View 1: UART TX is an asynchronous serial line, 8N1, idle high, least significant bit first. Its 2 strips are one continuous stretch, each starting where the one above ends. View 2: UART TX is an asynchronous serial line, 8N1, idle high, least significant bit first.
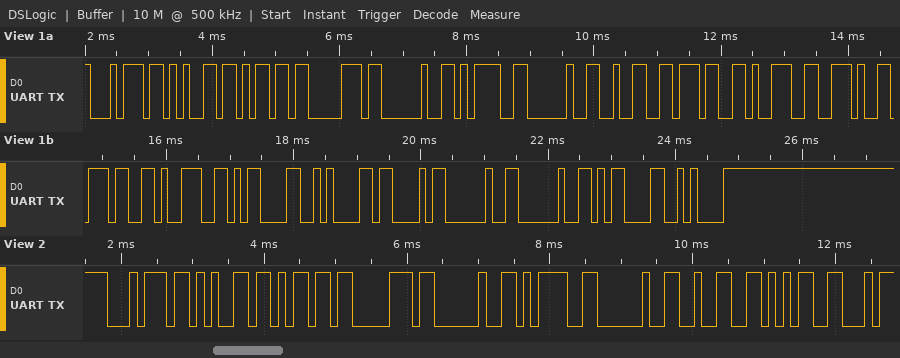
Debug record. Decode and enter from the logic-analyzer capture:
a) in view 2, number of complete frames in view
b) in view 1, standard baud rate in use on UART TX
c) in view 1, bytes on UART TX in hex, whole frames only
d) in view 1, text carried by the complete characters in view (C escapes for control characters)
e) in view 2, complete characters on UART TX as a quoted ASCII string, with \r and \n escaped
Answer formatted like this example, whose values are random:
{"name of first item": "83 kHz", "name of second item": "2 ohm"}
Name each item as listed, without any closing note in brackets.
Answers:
{"in view 2, number of complete frames in view": "9", "in view 1, standard baud rate in use on UART TX": "9600 baud", "in view 1, bytes on UART TX in hex, whole frames only": "0x74 0x65 0x6D 0x70 0x20 0x3D 0x20 0x32 0x37 0x39 0x2E 0x37 0x39 0x0D 0x0A 0x43 0x20 0x20 0x0D 0x0A", "in view 1, text carried by the complete characters in view": "\"temp = 279.79\\r\\nC  \\r\\n\"", "in view 2, complete characters on UART TX as a quoted ASCII string, with \\r and \\n escaped": "\"temp = 25\""}
